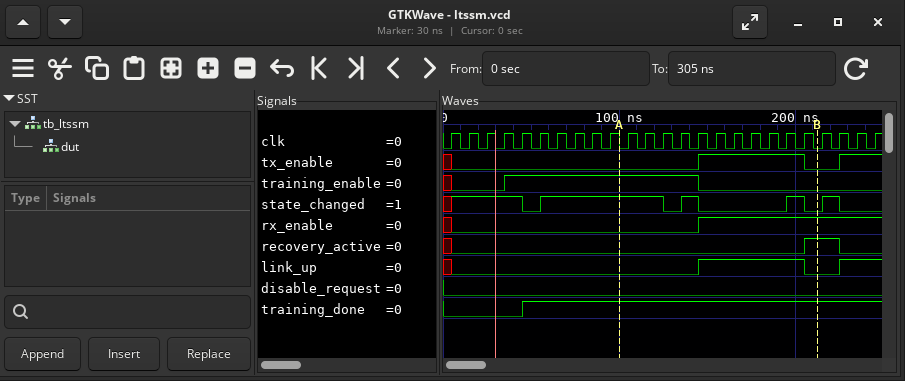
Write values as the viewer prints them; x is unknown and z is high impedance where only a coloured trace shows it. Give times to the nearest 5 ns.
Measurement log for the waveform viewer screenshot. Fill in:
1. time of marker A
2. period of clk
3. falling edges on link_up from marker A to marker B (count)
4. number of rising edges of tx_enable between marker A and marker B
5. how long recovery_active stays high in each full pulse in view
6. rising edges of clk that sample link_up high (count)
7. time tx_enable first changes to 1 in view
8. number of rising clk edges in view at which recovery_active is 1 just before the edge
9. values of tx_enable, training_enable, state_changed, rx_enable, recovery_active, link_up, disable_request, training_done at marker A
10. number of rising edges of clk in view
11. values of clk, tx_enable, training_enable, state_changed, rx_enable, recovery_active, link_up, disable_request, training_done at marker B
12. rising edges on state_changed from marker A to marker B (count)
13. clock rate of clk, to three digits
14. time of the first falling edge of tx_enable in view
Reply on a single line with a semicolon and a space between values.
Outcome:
100 ns; 10 ns; 1; 1; 20 ns; 8; 145 ns; 2; tx_enable=0, training_enable=1, state_changed=1, rx_enable=0, recovery_active=0, link_up=0, disable_request=0, training_done=1; 25; clk=0, tx_enable=0, training_enable=0, state_changed=0, rx_enable=1, recovery_active=1, link_up=0, disable_request=0, training_done=1; 2; 100 MHz; 205 ns
